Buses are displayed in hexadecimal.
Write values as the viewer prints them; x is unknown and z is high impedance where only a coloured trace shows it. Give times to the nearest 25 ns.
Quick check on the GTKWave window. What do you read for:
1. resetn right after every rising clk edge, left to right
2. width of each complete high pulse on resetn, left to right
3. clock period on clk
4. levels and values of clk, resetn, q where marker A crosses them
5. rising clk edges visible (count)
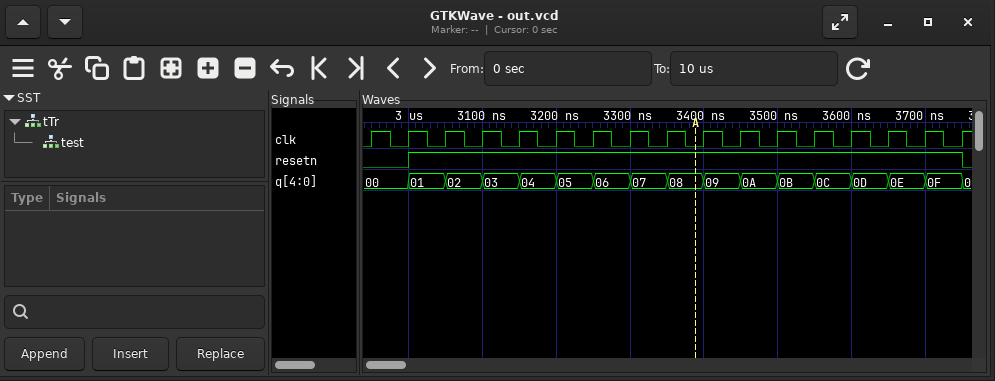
0 1 1 1 1 1 1 1 1 1 1 1 1 1 1 1 0
750 ns
50 ns
clk=0, resetn=1, q=08
17
